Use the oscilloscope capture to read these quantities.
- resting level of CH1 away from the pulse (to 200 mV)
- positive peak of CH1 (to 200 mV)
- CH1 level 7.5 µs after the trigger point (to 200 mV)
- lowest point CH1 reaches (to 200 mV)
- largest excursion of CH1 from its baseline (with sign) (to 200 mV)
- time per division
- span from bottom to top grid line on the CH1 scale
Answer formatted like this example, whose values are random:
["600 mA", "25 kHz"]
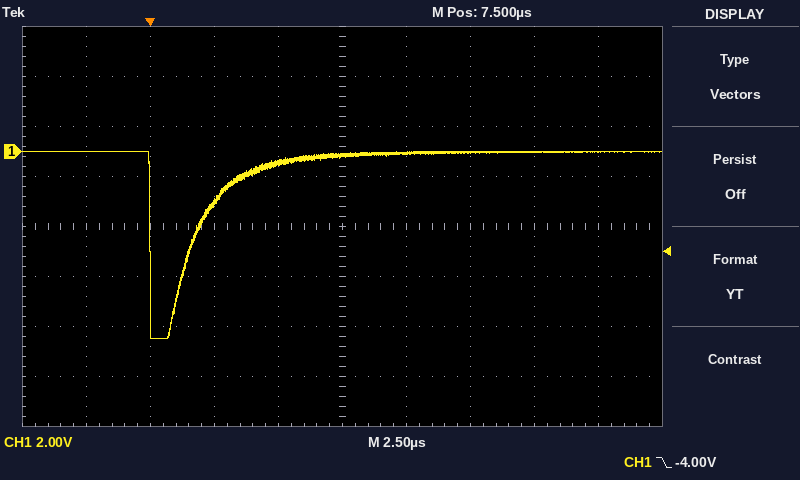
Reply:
["0.0 V", "0.0 V", "-200 mV", "-7.4 V", "-7.4 V", "2.5 µs", "16 V"]
